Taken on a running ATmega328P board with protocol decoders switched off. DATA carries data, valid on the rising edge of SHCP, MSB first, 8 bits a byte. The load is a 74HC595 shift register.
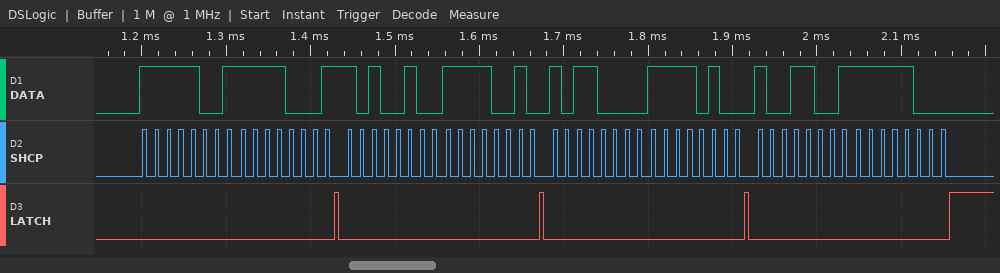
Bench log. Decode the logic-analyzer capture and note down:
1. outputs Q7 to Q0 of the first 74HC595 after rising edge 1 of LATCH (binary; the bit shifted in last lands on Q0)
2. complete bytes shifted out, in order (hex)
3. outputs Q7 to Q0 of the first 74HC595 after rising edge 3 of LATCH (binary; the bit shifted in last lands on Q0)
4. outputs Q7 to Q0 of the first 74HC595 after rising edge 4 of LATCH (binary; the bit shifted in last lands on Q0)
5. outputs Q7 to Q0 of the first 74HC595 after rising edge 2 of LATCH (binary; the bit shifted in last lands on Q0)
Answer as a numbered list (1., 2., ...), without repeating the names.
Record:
1. 11110001
2. 0xF9 0xF1 0xA4 0xF2 0xB0 0xF4 0x99 0xF8
3. 11110100
4. 11111000
5. 11110010
